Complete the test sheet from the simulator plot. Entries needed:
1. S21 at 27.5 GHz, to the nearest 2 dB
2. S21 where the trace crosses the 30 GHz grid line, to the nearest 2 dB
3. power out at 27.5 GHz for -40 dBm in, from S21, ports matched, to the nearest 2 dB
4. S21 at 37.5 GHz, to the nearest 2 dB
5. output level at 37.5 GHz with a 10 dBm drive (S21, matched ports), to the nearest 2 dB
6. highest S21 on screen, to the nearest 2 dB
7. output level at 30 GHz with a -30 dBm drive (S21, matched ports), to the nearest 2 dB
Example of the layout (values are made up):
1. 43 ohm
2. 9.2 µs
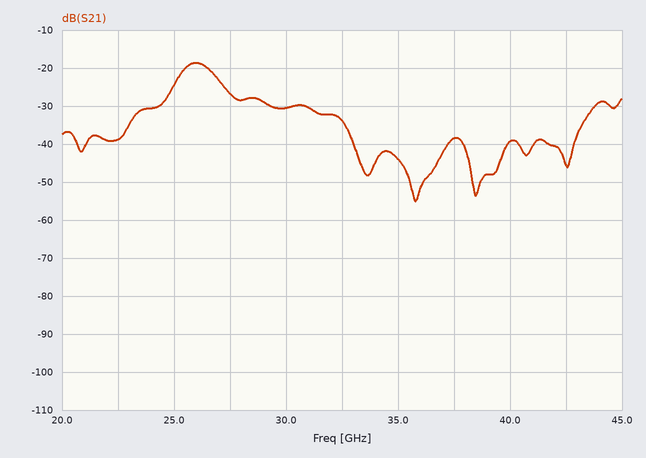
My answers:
1. -26 dB
2. -30 dB
3. -66 dBm
4. -38 dB
5. -28 dBm
6. -18 dB
7. -60 dBm
